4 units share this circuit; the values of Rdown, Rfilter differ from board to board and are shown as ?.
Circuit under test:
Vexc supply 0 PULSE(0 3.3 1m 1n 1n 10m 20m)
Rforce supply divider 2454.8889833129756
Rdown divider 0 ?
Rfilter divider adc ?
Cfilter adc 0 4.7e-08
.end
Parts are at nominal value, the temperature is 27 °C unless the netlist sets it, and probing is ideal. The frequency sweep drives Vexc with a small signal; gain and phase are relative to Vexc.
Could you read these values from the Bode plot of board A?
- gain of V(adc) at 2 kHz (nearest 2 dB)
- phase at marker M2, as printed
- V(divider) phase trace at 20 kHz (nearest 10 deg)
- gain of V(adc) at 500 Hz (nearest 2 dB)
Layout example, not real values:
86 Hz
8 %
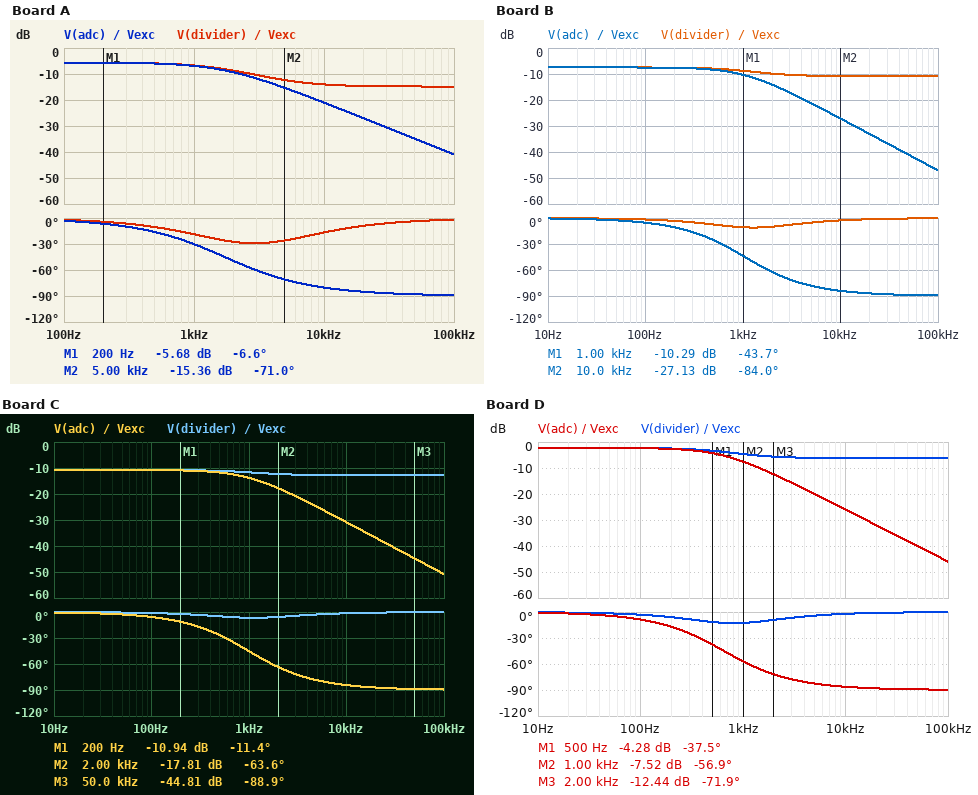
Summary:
-10 dB
-71.0 deg
-10 deg
-6 dB
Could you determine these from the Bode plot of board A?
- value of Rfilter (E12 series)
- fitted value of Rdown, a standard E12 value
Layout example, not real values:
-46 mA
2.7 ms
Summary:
680 Ω
2.7 kΩ
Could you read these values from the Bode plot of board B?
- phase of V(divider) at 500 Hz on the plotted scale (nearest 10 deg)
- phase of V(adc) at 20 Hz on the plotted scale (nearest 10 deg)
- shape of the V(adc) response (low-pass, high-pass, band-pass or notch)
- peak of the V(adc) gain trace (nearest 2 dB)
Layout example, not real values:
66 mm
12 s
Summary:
-10 deg
0 deg
low-pass
-8 dB
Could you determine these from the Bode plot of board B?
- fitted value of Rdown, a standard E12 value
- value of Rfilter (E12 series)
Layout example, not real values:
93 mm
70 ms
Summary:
1.8 kΩ
2.2 kΩ
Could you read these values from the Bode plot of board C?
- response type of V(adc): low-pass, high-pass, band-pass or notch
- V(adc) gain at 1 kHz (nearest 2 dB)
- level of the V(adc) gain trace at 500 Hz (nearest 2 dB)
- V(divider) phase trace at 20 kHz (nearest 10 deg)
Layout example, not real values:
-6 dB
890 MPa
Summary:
low-pass
-14 dB
-12 dB
0 deg
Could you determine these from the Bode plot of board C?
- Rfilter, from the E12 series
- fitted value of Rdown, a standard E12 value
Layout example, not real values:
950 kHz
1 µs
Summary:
2.7 kΩ
1 kΩ
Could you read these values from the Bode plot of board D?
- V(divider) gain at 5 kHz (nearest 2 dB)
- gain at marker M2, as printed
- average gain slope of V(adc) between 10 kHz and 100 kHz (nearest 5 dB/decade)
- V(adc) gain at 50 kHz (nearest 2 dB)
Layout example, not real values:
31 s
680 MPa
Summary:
-6 dB
-7.52 dB
-20 dB/decade
-40 dB
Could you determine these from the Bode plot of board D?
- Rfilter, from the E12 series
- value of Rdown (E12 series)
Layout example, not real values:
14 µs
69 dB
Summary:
3.3 kΩ
8.2 kΩ
